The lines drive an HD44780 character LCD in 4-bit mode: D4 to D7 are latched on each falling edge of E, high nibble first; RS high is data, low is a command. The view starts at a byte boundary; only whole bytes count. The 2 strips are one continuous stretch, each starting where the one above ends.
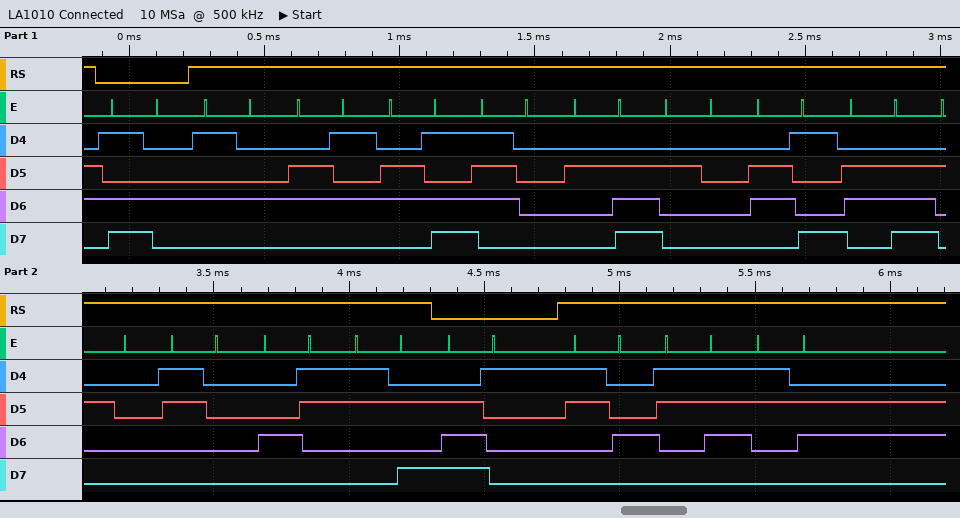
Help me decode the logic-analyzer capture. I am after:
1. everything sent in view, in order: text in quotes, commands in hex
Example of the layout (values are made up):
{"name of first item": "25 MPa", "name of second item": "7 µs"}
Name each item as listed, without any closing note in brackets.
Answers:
{"everything sent in view, in order: text in quotes, commands in hex": "0xD4 \"Temp. in 0C:\" 0xE1 \"476\""}
